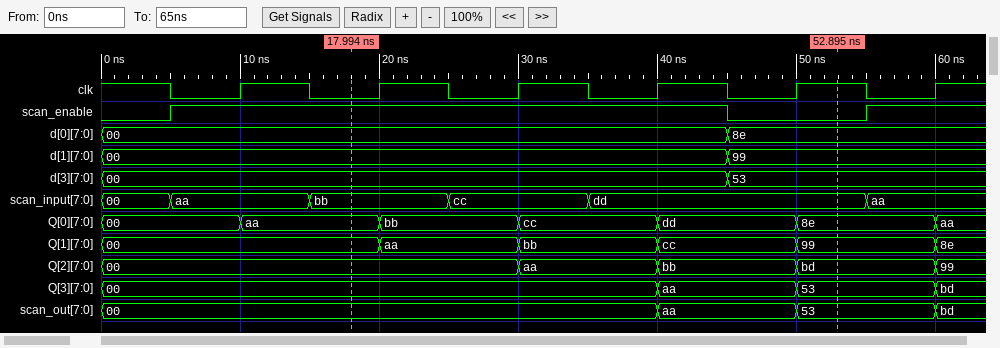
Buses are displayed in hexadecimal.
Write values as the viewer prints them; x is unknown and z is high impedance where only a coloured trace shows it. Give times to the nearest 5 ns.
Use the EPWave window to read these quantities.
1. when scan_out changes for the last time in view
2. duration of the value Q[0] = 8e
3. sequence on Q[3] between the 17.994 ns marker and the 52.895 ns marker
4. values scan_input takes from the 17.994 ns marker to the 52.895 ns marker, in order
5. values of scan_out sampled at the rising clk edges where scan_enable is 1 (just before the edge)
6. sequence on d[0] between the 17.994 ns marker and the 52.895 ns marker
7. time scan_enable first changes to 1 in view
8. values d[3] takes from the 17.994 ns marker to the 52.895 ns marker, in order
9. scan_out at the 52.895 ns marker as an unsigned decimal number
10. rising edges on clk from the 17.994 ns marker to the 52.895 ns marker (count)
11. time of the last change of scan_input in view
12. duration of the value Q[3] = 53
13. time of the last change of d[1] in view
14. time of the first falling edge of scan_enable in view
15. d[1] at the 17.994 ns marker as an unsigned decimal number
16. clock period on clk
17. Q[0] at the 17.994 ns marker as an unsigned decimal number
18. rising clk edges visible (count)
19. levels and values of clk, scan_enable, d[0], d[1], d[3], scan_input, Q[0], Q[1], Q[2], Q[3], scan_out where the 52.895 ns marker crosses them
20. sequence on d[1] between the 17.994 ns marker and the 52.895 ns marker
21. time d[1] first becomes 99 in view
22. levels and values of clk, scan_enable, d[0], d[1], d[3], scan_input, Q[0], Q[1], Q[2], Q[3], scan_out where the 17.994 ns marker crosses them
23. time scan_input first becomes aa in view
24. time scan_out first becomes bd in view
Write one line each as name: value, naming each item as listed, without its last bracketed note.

when scan_out changes for the last time in view: 60 ns
duration of the value Q[0] = 8e: 10 ns
sequence on Q[3] between the 17.994 ns marker and the 52.895 ns marker: 00, aa, 53
values scan_input takes from the 17.994 ns marker to the 52.895 ns marker, in order: bb, cc, dd
values of scan_out sampled at the rising clk edges where scan_enable is 1: 00, 00, 00, 00, 53
sequence on d[0] between the 17.994 ns marker and the 52.895 ns marker: 00, 8e
time scan_enable first changes to 1 in view: 5 ns
values d[3] takes from the 17.994 ns marker to the 52.895 ns marker, in order: 00, 53
scan_out at the 52.895 ns marker as an unsigned decimal number: 83
rising edges on clk from the 17.994 ns marker to the 52.895 ns marker: 4
time of the last change of scan_input in view: 55 ns
duration of the value Q[3] = 53: 10 ns
time of the last change of d[1] in view: 45 ns
time of the first falling edge of scan_enable in view: 45 ns
d[1] at the 17.994 ns marker as an unsigned decimal number: 0
clock period on clk: 10 ns
Q[0] at the 17.994 ns marker as an unsigned decimal number: 170
rising clk edges visible: 6
levels and values of clk, scan_enable, d[0], d[1], d[3], scan_input, Q[0], Q[1], Q[2], Q[3], scan_out where the 52.895 ns marker crosses them: clk=1, scan_enable=0, d[0]=8e, d[1]=99, d[3]=53, scan_input=dd, Q[0]=8e, Q[1]=99, Q[2]=bd, Q[3]=53, scan_out=53
sequence on d[1] between the 17.994 ns marker and the 52.895 ns marker: 00, 99
time d[1] first becomes 99 in view: 45 ns
levels and values of clk, scan_enable, d[0], d[1], d[3], scan_input, Q[0], Q[1], Q[2], Q[3], scan_out where the 17.994 ns marker crosses them: clk=0, scan_enable=1, d[0]=00, d[1]=00, d[3]=00, scan_input=bb, Q[0]=aa, Q[1]=00, Q[2]=00, Q[3]=00, scan_out=00
time scan_input first becomes aa in view: 5 ns
time scan_out first becomes bd in view: 60 ns
